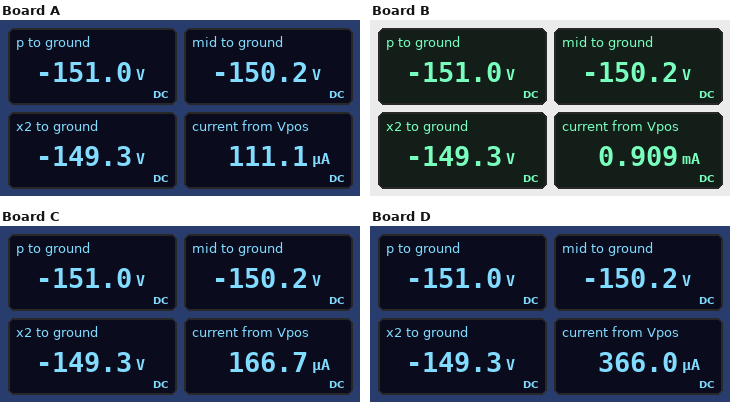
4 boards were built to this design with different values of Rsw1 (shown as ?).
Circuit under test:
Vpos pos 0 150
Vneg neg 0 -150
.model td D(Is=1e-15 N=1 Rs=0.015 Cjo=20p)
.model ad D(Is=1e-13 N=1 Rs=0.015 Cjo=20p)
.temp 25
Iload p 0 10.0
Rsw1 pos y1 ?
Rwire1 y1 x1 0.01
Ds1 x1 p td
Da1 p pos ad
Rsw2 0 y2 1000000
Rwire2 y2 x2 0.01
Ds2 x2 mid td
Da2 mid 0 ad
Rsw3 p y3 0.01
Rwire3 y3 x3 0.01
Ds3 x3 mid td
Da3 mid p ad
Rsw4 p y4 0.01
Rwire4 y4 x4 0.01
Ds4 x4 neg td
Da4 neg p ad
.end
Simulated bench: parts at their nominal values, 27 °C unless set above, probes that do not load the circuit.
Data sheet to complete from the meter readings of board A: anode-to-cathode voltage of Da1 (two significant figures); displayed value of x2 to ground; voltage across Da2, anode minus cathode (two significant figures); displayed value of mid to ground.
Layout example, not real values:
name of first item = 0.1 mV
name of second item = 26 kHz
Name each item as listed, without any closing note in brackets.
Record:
anode-to-cathode voltage of Da1 = -300 V
displayed value of x2 to ground = -149.3 V
voltage across Da2, anode minus cathode = -150 V
displayed value of mid to ground = -150.2 V
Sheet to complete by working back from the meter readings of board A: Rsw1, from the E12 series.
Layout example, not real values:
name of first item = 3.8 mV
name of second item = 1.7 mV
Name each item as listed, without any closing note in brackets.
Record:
Rsw1, from the E12 series = 2.7 MΩ
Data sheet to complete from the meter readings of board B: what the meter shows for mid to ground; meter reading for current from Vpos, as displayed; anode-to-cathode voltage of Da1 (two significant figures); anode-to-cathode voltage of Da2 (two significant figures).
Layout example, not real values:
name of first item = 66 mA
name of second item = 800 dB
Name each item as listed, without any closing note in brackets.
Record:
what the meter shows for mid to ground = -150.2 V
meter reading for current from Vpos, as displayed = 0.909 mA
anode-to-cathode voltage of Da1 = -300 V
anode-to-cathode voltage of Da2 = -150 V
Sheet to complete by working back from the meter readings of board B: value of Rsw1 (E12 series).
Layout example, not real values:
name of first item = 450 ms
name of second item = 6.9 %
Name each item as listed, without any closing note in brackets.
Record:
value of Rsw1 = 330 kΩ
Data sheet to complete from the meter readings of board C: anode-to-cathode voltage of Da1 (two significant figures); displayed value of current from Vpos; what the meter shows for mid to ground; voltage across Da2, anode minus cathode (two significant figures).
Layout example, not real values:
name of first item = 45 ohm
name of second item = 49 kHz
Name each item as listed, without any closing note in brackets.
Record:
anode-to-cathode voltage of Da1 = -300 V
displayed value of current from Vpos = 166.7 µA
what the meter shows for mid to ground = -150.2 V
voltage across Da2, anode minus cathode = -150 V
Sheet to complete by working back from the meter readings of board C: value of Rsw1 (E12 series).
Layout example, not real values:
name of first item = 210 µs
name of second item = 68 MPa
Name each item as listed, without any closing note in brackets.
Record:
value of Rsw1 = 1.8 MΩ
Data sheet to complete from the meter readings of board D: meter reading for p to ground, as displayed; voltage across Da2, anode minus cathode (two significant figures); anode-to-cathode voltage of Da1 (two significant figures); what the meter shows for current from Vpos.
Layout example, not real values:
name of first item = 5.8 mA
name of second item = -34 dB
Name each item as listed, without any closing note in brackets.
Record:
meter reading for p to ground, as displayed = -151.0 V
voltage across Da2, anode minus cathode = -150 V
anode-to-cathode voltage of Da1 = -300 V
what the meter shows for current from Vpos = 366.0 µA
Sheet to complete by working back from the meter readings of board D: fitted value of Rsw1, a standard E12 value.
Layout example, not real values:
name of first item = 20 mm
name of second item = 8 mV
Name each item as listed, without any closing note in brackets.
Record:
fitted value of Rsw1, a standard E12 value = 820 kΩ
